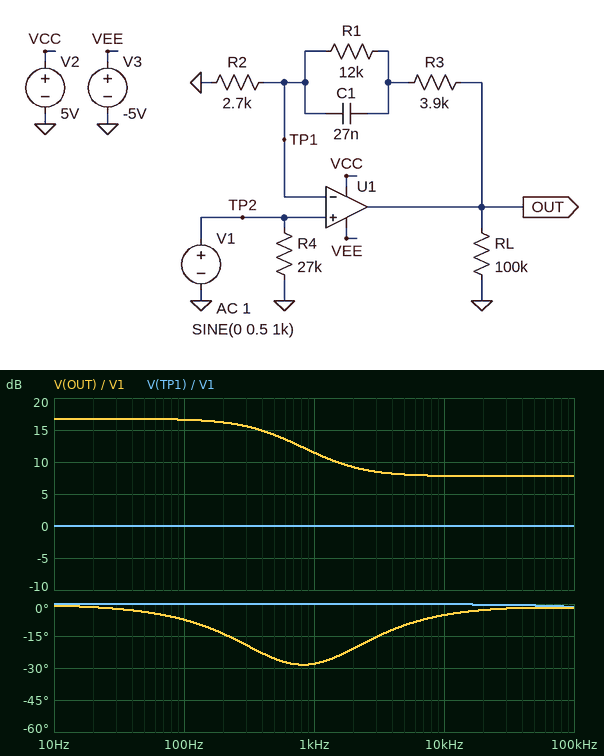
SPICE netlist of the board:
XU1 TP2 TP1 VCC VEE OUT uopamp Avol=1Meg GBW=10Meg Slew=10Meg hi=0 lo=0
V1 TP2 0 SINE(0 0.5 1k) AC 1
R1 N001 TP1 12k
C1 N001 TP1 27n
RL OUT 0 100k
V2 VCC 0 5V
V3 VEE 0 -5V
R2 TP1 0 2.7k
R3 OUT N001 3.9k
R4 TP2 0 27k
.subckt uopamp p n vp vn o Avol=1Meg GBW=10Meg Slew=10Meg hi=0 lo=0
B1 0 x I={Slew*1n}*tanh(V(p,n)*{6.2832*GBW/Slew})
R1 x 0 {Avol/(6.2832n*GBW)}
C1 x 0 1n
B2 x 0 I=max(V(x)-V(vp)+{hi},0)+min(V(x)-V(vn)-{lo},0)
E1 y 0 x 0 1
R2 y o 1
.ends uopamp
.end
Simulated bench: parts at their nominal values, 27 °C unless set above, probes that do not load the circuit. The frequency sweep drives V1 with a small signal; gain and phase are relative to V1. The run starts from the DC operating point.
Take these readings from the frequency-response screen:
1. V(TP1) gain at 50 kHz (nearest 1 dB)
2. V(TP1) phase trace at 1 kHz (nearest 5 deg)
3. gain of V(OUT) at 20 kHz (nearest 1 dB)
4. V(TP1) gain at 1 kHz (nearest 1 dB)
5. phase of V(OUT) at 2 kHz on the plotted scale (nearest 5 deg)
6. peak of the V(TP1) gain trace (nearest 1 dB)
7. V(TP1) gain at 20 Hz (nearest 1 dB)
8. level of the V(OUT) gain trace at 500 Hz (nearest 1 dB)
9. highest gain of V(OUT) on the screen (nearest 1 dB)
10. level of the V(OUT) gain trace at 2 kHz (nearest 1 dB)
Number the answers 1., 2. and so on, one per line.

1. 0 dB
2. 0 deg
3. 8 dB
4. 0 dB
5. -20 deg
6. 0 dB
7. 0 dB
8. 14 dB
9. 17 dB
10. 9 dB
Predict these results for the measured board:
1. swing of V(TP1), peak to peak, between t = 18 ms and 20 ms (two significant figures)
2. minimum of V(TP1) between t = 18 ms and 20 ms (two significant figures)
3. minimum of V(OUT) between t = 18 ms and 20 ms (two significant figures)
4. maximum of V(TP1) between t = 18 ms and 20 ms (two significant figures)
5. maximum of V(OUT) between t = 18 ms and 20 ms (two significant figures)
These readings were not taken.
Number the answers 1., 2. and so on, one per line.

1. 1.0 V
2. -500 mV
3. -1.9 V
4. 500 mV
5. 1.9 V
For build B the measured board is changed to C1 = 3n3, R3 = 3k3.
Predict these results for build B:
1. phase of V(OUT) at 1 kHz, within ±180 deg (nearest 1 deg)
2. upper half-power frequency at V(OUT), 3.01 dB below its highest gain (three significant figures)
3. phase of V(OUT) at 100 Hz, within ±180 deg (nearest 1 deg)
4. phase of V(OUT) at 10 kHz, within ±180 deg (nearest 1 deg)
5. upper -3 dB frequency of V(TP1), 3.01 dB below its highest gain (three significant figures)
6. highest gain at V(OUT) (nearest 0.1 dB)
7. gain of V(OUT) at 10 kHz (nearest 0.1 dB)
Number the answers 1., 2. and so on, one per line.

1. -9 deg
2. 4.55 kHz
3. -1 deg
4. -29 deg
5. 4.49 MHz
6. 16.5 dB
7. 10.2 dB
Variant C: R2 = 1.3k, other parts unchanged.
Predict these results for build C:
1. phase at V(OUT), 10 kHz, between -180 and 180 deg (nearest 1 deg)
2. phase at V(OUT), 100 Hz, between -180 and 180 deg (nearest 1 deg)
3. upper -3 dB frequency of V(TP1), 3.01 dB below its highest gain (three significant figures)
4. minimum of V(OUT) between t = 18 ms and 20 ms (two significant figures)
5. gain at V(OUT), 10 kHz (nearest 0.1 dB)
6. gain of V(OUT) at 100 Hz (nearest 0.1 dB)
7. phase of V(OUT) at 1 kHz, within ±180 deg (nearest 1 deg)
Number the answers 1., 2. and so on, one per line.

1. -7 deg
2. -8 deg
3. 2.50 MHz
4. -3.4 V
5. 12.1 dB
6. 22.3 dB
7. -32 deg
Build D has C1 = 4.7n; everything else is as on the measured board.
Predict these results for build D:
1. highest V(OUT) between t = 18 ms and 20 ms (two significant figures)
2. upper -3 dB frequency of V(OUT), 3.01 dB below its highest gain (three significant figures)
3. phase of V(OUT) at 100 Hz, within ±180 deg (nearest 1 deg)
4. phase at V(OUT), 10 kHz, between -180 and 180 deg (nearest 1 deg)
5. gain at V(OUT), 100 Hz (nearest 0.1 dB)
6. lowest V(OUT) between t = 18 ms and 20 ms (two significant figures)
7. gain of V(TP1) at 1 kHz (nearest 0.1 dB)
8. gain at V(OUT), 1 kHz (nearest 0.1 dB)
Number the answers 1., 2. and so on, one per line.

1. 3.3 V
2. 3.26 kHz
3. -1 deg
4. -23 deg
5. 16.8 dB
6. -3.3 V
7. 0 dB
8. 16.3 dB
